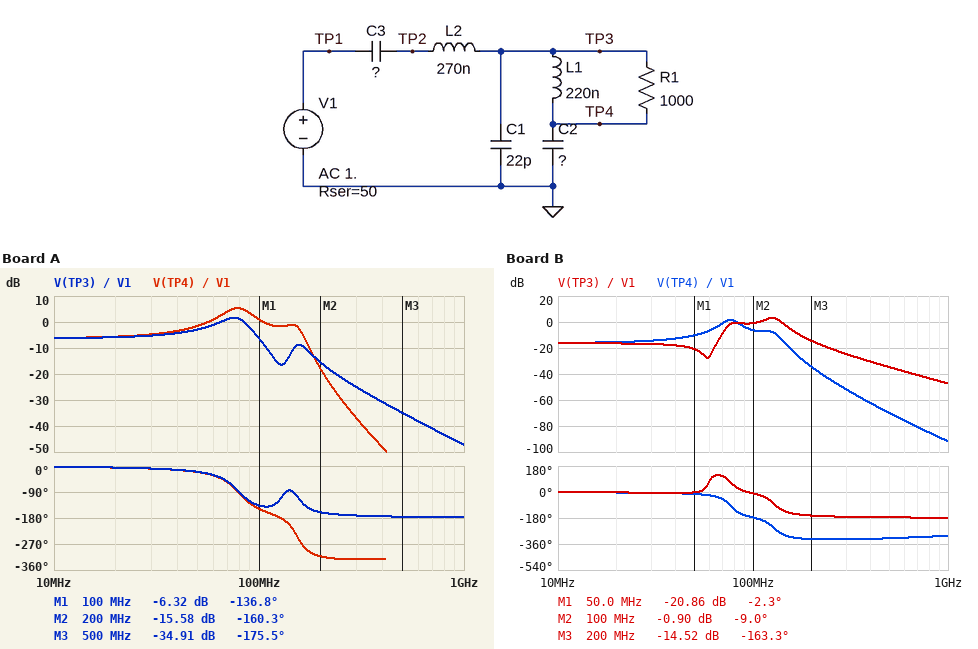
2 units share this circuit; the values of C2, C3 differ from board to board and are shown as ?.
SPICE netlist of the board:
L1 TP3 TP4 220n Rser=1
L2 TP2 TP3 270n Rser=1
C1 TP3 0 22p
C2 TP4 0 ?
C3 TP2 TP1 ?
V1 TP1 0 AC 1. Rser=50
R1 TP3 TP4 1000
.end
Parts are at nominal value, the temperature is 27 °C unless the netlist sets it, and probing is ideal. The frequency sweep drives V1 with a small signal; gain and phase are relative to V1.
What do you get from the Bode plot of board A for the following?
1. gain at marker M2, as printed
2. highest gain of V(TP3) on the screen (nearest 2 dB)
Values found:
-15.58 dB
2 dB
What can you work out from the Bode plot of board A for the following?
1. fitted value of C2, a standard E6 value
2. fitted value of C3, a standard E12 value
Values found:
6.8 pF
27 pF
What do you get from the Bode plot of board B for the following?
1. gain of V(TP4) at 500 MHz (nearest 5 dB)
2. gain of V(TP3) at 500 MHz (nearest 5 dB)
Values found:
-70 dB
-35 dB
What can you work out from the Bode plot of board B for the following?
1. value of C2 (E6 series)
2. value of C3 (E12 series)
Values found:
33 pF
10 pF
